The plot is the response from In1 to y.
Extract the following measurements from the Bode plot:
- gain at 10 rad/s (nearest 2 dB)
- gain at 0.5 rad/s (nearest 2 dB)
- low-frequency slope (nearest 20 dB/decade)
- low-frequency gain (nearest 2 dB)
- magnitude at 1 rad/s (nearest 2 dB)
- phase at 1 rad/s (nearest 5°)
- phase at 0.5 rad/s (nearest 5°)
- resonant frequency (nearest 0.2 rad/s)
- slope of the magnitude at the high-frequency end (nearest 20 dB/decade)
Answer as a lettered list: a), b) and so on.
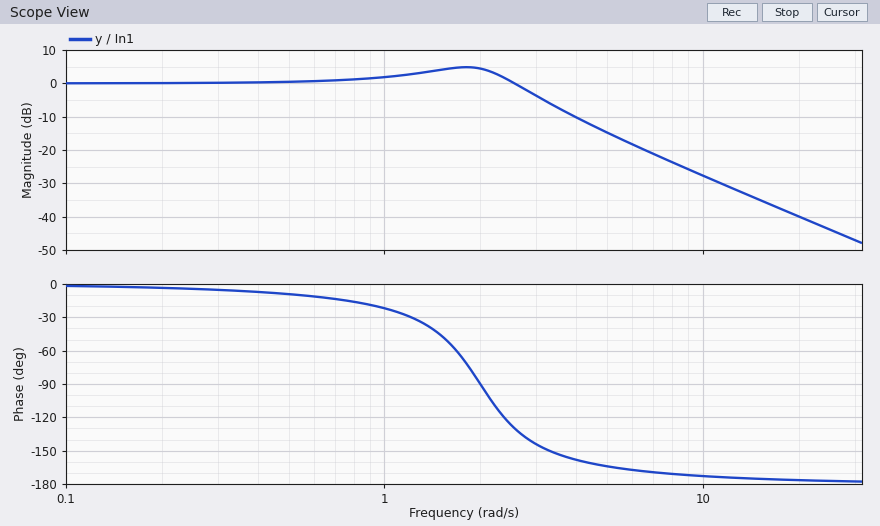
a) -28 dB
b) 0 dB
c) 0 dB/decade
d) 0 dB
e) 2 dB
f) -20°
g) -10°
h) 1.8 rad/s
i) -40 dB/decade
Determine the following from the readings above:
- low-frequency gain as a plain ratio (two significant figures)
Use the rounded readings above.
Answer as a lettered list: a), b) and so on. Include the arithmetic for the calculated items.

a) 10^(0 / 20) = 1.0
